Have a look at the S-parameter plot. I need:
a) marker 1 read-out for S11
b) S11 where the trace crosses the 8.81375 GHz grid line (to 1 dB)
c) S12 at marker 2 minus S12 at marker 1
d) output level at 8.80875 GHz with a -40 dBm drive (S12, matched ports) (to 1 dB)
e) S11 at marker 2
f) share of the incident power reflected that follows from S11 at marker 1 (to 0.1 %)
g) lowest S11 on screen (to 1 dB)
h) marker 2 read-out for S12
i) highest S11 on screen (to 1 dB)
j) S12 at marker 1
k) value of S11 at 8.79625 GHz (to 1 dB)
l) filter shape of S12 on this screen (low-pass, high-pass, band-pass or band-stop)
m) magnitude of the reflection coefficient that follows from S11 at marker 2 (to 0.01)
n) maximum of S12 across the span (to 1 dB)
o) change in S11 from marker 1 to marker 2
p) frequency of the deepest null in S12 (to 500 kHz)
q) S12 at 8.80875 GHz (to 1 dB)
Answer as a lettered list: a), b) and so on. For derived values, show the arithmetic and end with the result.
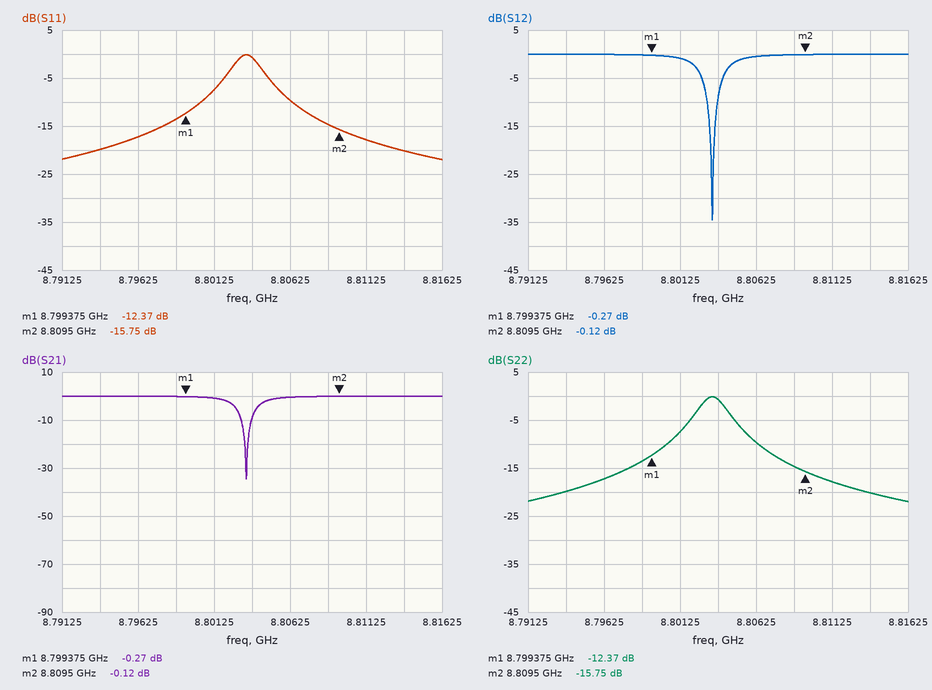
a) -12.37 dB
b) -20 dB
c) -0.12 − (-0.27) = 0.15 dB
d) -40 dBm + (0 dB) = -40 dBm
e) -15.75 dB
f) 10^(-12.37/10) ≈ 5.8 %
g) -22 dB
h) -0.12 dB
i) 0 dB
j) -0.27 dB
k) -17 dB
l) band-stop
m) 10^(-15.75/20) ≈ 0.16
n) 0 dB
o) -15.75 − (-12.37) = -3.38 dB
p) 8.8035 GHz
q) 0 dB
